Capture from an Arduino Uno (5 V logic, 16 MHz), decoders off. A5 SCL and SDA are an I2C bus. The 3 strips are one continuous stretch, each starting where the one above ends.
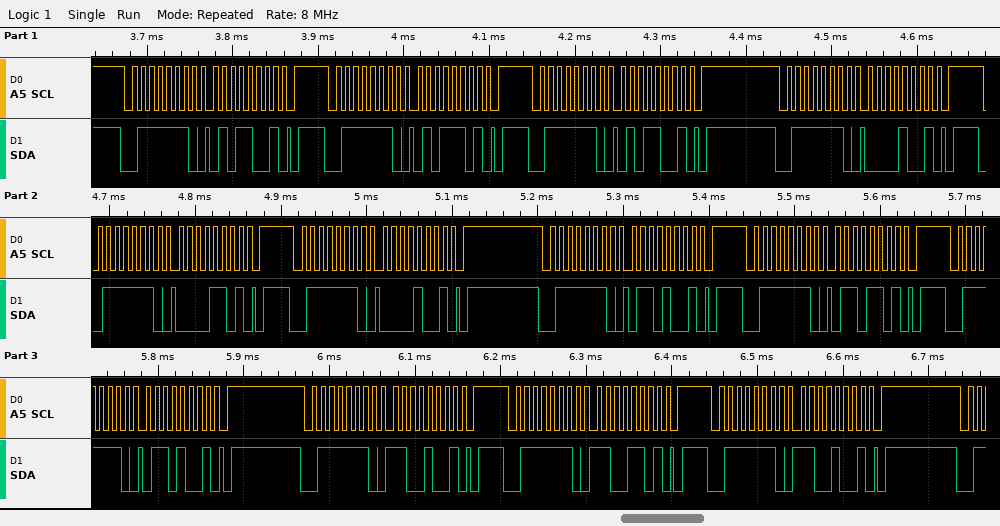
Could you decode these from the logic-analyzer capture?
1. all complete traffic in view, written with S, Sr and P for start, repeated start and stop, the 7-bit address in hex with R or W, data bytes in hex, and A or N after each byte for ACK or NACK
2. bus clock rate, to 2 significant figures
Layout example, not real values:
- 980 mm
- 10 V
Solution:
- S 3FW A 59 A P S 3FW A 5D A P S 3FW A 59 A P S 3FW A 09 A P S 3FW A 0D A P S 3FW A 09 A P S 3FW A 69 A P S 3FW A 6D A P S 3FW A 69 A P S 3FW A C9 A P S 3FW A CD A P S 3FW A C9 A P
- 100 kHz
